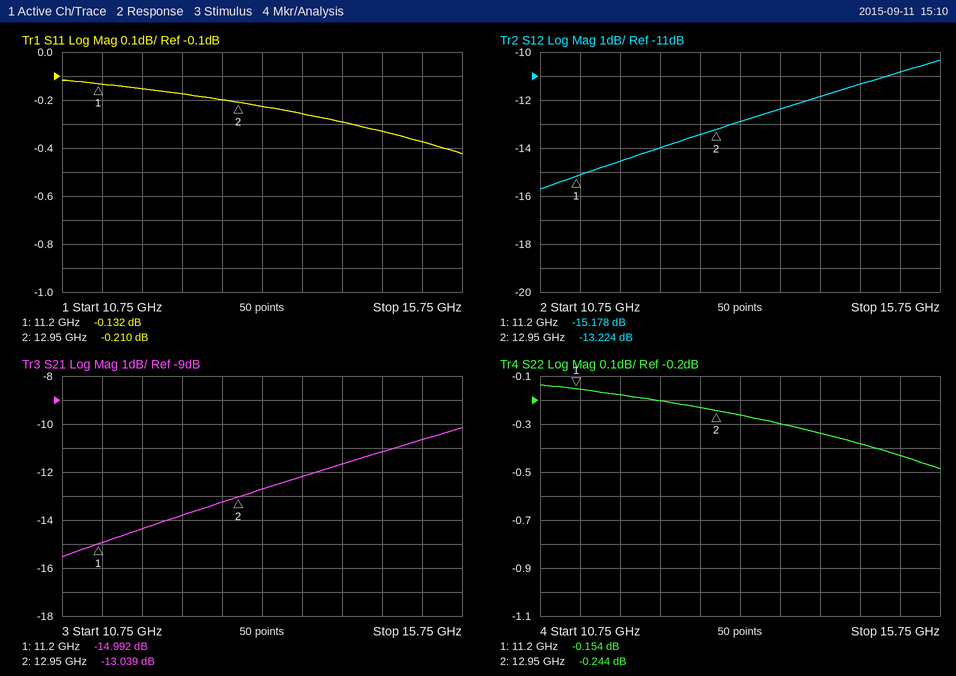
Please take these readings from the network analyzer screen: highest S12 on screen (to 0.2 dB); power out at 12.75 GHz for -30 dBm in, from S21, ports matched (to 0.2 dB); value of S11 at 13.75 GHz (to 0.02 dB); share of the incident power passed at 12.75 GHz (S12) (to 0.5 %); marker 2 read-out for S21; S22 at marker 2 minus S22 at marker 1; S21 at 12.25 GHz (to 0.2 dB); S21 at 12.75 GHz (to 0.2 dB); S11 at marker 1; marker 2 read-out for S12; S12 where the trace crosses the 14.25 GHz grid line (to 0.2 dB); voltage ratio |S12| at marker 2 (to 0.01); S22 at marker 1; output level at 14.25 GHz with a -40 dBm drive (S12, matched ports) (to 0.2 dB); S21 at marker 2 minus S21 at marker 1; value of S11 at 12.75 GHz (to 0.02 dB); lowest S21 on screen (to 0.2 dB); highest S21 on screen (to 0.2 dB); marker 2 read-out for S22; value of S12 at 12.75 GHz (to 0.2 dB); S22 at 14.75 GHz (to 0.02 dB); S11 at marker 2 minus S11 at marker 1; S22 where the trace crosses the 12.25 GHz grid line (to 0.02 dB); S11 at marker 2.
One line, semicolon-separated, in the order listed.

-10.4 dB; -43.2 dBm; -0.26 dB; 4.5 %; -13.039 dB; -0.090 dB; -13.8 dB; -13.2 dB; -0.132 dB; -13.224 dB; -11.8 dB; 0.22; -0.154 dB; -51.8 dBm; 1.953 dB; -0.20 dB; -15.6 dB; -10.2 dB; -0.244 dB; -13.4 dB; -0.38 dB; -0.078 dB; -0.20 dB; -0.210 dB
